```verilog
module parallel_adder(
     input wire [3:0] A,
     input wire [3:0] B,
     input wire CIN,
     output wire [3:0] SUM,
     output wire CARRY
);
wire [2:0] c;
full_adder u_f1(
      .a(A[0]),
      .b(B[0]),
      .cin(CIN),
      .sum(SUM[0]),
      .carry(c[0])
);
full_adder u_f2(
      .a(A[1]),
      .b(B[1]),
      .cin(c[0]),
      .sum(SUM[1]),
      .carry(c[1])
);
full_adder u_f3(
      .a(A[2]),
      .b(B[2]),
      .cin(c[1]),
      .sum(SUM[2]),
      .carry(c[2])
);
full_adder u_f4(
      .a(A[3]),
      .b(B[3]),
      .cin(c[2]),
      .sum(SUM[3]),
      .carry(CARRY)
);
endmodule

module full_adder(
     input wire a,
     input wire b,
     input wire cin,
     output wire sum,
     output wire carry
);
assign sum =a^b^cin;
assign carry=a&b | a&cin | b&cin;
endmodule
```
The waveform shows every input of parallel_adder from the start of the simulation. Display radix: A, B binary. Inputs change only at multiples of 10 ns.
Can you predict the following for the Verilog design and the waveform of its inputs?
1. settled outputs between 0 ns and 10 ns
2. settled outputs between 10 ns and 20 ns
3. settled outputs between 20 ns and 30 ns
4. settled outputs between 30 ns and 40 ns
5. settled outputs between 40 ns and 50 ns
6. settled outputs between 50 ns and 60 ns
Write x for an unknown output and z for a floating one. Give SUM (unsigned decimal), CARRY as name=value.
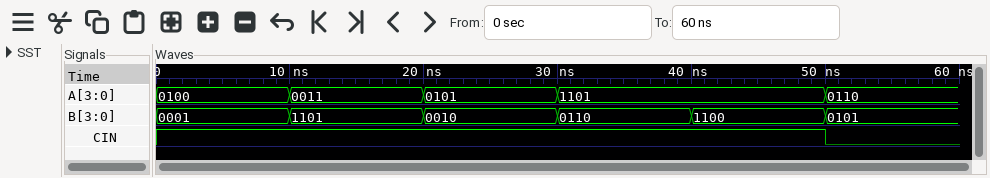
SUM=6, CARRY=0
SUM=1, CARRY=1
SUM=8, CARRY=0
SUM=4, CARRY=1
SUM=10, CARRY=1
SUM=11, CARRY=0
